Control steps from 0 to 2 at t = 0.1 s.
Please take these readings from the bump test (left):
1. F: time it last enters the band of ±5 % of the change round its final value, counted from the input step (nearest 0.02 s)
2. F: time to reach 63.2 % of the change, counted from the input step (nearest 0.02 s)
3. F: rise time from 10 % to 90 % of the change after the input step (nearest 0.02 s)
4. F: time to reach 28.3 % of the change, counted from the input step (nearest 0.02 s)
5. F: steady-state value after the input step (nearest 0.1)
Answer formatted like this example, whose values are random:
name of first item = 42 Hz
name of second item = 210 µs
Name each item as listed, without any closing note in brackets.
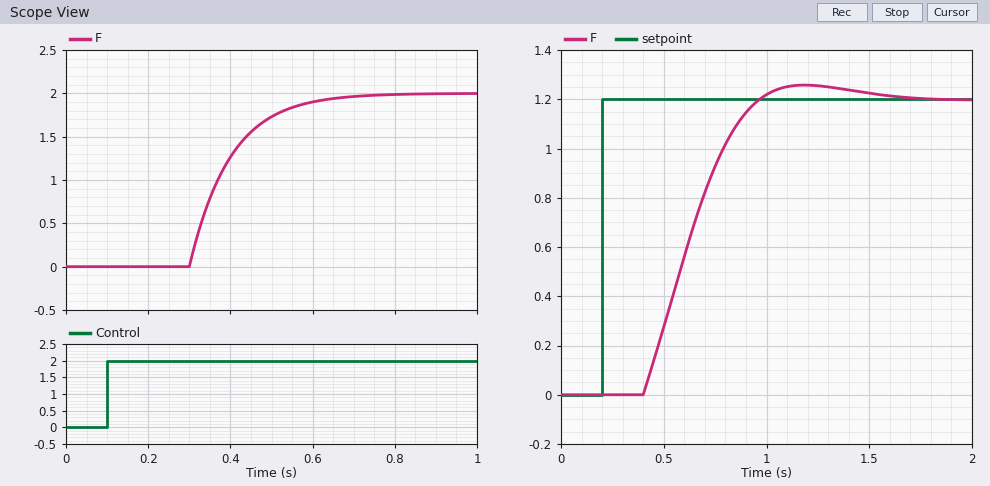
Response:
F: time it last enters the band of ±5 % of the change round its final value, counted from the input step = 0.50 s
F: time to reach 63.2 % of the change, counted from the input step = 0.30 s
F: rise time from 10 % to 90 % of the change after the input step = 0.22 s
F: time to reach 28.3 % of the change, counted from the input step = 0.24 s
F: steady-state value after the input step = 2.0
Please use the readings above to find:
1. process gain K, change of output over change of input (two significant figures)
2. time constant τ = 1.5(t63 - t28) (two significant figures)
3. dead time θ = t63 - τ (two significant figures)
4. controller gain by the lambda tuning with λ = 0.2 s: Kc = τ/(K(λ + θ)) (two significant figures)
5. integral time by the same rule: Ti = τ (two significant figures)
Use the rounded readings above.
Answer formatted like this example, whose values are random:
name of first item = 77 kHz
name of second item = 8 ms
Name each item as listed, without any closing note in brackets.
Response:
process gain K, change of output over change of input = 1.0
time constant τ = 1.5(t63 - t28) = 0.090 s
dead time θ = t63 - τ = 0.21 s
controller gain by the lambda tuning with λ = 0.2 s: Kc = τ/(K(λ + θ)) = 0.22
integral time by the same rule: Ti = τ = 0.090 s
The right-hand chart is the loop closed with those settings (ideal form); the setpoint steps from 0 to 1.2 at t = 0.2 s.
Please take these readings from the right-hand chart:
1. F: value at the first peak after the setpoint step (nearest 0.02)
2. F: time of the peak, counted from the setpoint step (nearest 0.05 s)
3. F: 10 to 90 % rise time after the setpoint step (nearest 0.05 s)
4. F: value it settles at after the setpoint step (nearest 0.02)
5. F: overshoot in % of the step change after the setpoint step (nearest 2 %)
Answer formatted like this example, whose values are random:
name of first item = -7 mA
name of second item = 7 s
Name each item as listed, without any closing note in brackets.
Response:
F: value at the first peak after the setpoint step = 1.26
F: time of the peak, counted from the setpoint step = 1.00 s
F: 10 to 90 % rise time after the setpoint step = 0.40 s
F: value it settles at after the setpoint step = 1.20
F: overshoot in % of the step change after the setpoint step = 4 %
